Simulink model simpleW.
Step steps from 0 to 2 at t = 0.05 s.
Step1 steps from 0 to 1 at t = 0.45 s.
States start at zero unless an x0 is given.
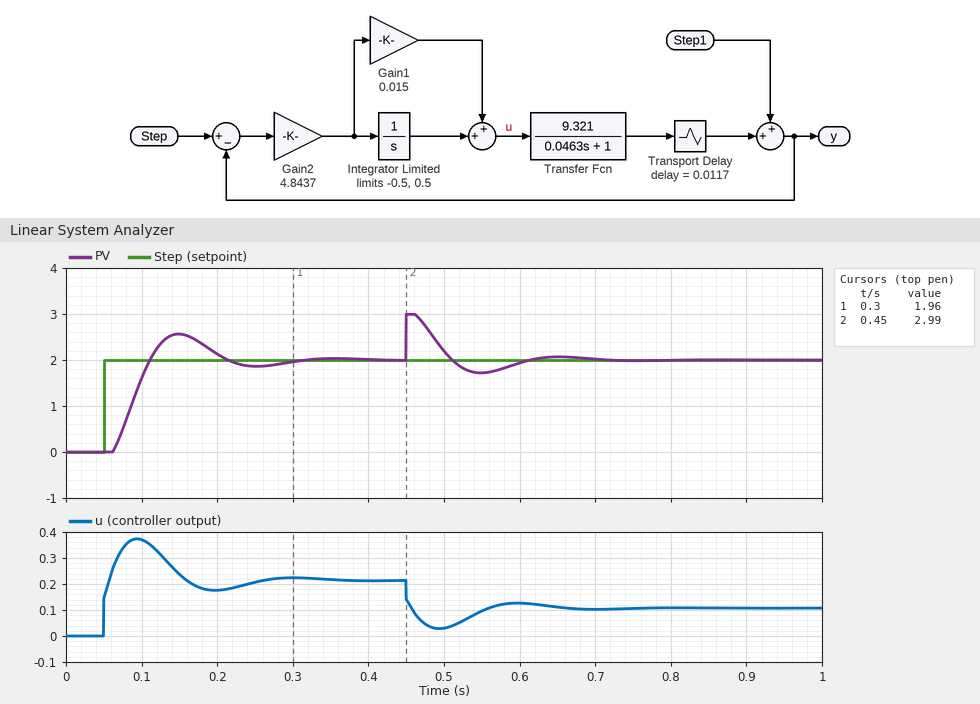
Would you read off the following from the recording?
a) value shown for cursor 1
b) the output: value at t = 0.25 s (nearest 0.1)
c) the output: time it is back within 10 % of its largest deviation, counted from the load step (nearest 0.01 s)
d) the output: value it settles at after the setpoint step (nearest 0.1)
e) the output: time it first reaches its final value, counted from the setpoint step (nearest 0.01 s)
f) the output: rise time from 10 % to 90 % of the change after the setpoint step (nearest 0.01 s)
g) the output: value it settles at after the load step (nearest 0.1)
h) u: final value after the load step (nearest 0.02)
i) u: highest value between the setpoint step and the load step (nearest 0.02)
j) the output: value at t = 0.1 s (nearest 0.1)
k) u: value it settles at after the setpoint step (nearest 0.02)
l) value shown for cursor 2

1.96
1.9
0.14 s
2.0
0.06 s
0.04 s
2.0
0.10
0.38
1.6
0.22
2.99
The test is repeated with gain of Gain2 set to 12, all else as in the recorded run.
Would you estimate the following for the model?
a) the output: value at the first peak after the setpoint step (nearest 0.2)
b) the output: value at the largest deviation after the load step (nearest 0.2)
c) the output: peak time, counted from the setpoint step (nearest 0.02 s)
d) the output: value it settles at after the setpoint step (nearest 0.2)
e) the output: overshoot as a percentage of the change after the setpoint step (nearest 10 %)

3.0
3.0
0.06 s
2.0
50 %
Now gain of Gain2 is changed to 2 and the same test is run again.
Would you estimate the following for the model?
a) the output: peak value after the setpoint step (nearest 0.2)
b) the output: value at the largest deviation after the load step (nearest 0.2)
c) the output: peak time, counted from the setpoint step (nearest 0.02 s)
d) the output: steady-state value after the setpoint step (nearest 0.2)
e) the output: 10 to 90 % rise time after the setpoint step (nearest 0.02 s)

2.2
3.0
0.18 s
2.0
0.08 s
